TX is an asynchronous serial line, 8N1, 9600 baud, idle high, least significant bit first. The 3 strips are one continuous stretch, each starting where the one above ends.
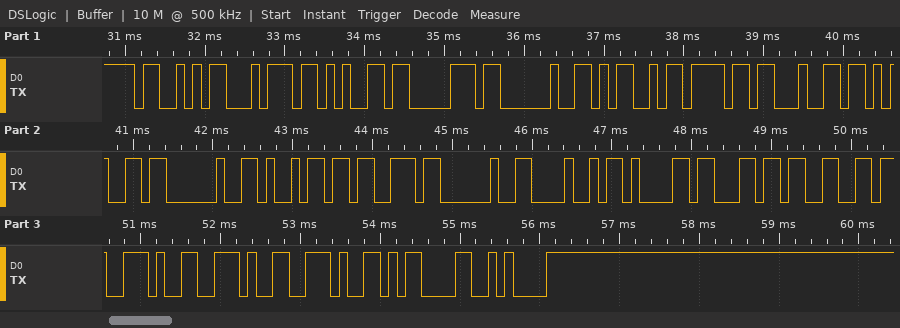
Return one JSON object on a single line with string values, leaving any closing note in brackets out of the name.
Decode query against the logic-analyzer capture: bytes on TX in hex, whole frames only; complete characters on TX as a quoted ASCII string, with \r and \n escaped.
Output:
{"bytes on TX in hex, whole frames only": "53 74 65 70 20 4D 6F 64 65 20 69 73 20 48 61 6C 66 2E 2E 2E 0D 0A", "complete characters on TX as a quoted ASCII string, with \\r and \\n escaped": "\"Step Mode is Half...\\r\\n\""}
